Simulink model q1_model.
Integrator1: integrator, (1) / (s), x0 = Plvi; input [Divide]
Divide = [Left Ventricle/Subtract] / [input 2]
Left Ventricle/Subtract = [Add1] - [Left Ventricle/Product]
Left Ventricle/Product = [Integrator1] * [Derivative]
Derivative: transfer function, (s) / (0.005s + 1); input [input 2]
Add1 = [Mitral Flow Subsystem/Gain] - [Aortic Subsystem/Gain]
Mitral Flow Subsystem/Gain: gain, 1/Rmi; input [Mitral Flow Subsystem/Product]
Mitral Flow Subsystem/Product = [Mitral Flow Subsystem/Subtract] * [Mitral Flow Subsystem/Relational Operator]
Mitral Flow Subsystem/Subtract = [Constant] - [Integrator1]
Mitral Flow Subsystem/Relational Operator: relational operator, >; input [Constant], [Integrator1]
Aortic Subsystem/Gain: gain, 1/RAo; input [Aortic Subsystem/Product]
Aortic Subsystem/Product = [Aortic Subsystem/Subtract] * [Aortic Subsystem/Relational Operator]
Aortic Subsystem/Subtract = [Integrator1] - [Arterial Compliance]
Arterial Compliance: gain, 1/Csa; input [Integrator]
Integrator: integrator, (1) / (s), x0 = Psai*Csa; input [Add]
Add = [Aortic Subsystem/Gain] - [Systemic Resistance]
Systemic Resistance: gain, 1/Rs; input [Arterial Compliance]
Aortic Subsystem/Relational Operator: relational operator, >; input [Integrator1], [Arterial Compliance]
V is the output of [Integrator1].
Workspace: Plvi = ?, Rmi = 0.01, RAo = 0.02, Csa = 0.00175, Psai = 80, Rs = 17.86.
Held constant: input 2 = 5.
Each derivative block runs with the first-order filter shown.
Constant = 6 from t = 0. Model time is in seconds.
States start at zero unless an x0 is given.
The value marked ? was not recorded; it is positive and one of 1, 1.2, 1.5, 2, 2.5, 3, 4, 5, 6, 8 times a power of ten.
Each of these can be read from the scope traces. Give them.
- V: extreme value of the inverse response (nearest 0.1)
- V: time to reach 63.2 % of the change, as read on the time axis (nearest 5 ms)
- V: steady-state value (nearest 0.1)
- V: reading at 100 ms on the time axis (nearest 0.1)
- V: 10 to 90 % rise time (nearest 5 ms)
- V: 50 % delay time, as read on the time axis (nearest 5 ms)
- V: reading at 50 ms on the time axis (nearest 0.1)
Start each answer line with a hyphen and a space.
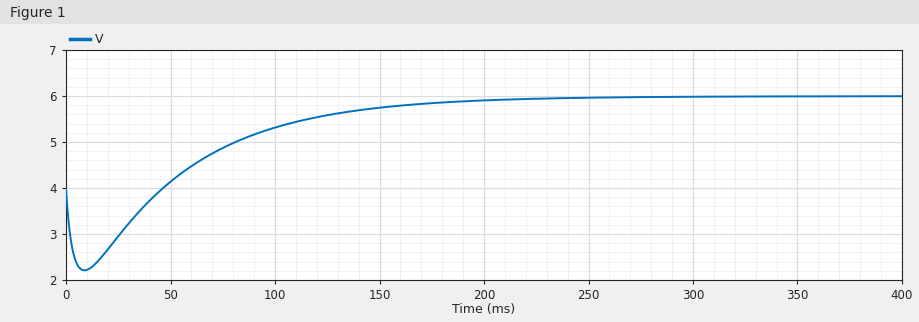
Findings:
- 2.2
- 95 ms
- 6.0
- 5.3
- 110 ms
- 80 ms
- 4.1
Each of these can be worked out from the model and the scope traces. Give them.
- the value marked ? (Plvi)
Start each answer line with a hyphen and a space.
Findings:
- 4
